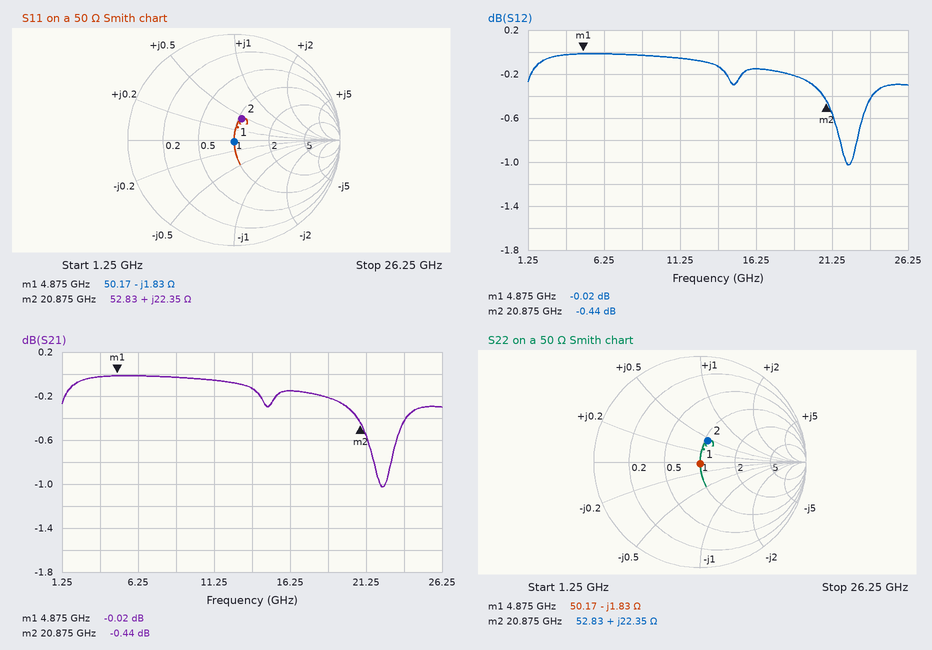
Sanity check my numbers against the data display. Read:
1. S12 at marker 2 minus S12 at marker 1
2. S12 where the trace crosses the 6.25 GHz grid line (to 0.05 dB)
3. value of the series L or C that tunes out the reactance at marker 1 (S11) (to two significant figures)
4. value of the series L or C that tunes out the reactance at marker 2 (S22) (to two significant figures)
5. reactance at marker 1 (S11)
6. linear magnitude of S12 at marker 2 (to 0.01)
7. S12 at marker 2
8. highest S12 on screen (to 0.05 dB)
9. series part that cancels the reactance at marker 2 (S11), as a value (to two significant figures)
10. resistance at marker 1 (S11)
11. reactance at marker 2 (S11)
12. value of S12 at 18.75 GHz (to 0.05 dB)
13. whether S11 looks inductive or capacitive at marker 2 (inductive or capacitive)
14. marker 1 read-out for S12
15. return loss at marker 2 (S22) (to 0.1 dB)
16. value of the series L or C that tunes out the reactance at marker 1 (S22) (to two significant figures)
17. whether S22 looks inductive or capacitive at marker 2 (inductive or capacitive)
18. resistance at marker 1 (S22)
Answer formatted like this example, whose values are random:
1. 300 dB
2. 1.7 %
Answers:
1. -0.42 dB
2. 0.00 dB
3. 60 pH
4. 340 fF
5. -1.83 Ω
6. 0.95
7. -0.44 dB
8. 0.00 dB
9. 340 fF
10. 50.17 Ω
11. +22.35 Ω
12. -0.20 dB
13. inductive
14. -0.02 dB
15. 13.4 dB
16. 60 pH
17. inductive
18. 50.17 Ω
